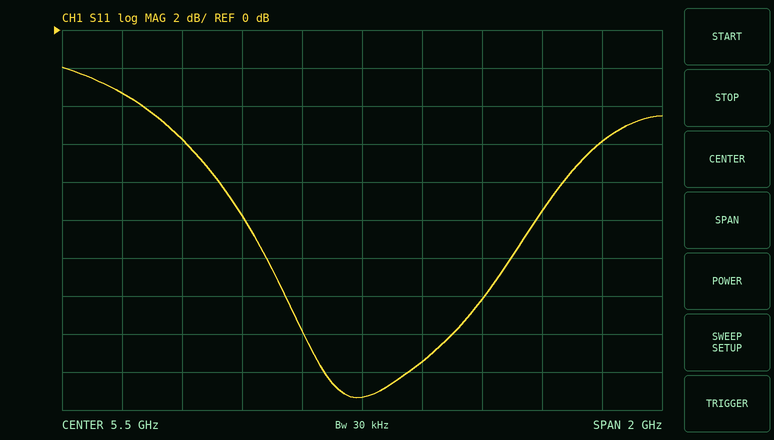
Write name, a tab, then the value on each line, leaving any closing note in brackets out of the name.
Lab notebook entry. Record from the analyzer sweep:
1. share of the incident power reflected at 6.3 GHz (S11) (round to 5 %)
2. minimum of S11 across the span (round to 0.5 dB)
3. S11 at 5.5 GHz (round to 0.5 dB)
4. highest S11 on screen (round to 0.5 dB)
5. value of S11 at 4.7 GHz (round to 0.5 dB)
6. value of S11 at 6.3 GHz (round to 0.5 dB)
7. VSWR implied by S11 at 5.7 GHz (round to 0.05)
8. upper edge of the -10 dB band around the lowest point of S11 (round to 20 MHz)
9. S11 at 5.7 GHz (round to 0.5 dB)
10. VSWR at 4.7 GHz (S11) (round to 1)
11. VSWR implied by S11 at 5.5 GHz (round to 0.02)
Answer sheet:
share of the incident power reflected at 6.3 GHz (S11)	25 %
minimum of S11 across the span	-19.5 dB
S11 at 5.5 GHz	-19.5 dB
highest S11 on screen	-2.0 dB
value of S11 at 4.7 GHz	-3.5 dB
value of S11 at 6.3 GHz	-6.0 dB
VSWR implied by S11 at 5.7 GHz	1.30
upper edge of the -10 dB band around the lowest point of S11	6.08 GHz
S11 at 5.7 GHz	-17.5 dB
VSWR at 4.7 GHz (S11)	5
VSWR implied by S11 at 5.5 GHz	1.24
